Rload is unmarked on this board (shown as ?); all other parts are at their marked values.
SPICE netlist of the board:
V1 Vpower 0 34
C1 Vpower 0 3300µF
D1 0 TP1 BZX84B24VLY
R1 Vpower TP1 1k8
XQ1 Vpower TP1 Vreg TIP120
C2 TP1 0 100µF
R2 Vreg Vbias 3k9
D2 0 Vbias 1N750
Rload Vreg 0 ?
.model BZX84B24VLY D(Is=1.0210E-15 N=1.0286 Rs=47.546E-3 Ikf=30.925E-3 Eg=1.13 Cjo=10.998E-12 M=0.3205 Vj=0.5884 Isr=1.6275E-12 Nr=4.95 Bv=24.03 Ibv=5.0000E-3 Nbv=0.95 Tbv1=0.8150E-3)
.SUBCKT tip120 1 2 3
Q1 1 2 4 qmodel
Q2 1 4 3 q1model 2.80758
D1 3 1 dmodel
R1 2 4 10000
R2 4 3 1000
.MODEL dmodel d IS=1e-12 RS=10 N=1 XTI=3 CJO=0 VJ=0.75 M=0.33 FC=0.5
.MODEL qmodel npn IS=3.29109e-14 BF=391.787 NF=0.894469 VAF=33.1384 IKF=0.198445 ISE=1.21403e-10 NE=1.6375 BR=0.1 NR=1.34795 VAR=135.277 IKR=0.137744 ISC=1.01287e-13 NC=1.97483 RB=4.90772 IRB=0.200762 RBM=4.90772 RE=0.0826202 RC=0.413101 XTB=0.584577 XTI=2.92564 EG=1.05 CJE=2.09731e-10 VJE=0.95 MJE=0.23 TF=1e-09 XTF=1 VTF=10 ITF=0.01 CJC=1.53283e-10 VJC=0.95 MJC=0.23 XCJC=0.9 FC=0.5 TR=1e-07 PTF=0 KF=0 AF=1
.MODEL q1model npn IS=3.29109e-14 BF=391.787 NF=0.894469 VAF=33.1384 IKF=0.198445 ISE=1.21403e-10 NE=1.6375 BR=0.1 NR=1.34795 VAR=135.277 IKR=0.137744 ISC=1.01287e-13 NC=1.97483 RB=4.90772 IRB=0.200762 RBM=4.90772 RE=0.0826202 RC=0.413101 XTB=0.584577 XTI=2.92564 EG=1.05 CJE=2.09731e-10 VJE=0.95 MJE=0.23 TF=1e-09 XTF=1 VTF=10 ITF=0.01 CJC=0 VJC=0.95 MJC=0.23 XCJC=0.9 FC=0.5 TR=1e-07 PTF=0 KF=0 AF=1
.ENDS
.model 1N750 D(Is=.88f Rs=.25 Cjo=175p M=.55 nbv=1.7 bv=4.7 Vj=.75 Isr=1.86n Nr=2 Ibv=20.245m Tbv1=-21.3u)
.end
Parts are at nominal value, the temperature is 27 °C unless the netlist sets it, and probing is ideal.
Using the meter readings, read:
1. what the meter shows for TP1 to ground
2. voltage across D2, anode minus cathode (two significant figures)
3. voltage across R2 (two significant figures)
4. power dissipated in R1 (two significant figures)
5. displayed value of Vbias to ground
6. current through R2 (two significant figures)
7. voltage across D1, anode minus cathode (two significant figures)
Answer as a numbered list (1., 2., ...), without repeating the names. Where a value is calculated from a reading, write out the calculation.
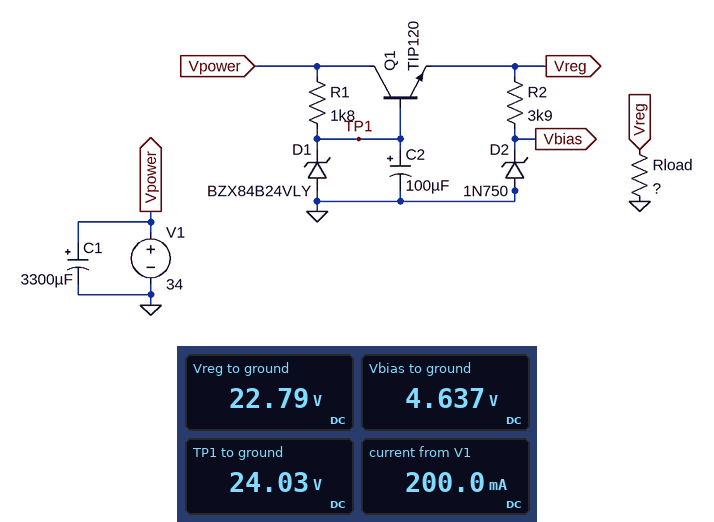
1. 24.03 V
2. 0 V - 4.637 V = -4.6 V
3. 22.79 V - 4.637 V = 18 V
4. (34 V - 24.03 V)^2 / 1.8 kΩ = 55 mW
5. 4.637 V
6. (22.79 V - 4.637 V) / 3.9 kΩ = 4.7 mA
7. 0 V - 24.03 V = -24 V
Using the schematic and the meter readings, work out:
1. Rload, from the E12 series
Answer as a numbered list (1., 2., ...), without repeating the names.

1. 120 Ω
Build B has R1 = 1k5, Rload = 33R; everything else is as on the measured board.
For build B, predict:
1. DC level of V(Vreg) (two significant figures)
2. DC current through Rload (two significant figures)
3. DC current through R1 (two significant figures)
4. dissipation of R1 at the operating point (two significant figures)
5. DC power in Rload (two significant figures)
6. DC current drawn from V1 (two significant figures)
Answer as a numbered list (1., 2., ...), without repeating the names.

1. 23 V
2. 690 mA
3. 6.6 mA
4. 66 mW
5. 16 W
6. 700 mA
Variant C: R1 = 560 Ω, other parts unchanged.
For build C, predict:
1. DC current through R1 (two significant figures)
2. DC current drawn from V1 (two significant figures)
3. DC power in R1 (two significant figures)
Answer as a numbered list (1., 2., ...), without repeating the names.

1. 18 mA
2. 210 mA
3. 180 mW
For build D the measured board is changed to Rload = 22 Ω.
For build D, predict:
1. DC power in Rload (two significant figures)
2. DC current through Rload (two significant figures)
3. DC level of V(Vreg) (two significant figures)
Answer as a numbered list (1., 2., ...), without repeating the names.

1. 23 W
2. 1.0 A
3. 23 V
